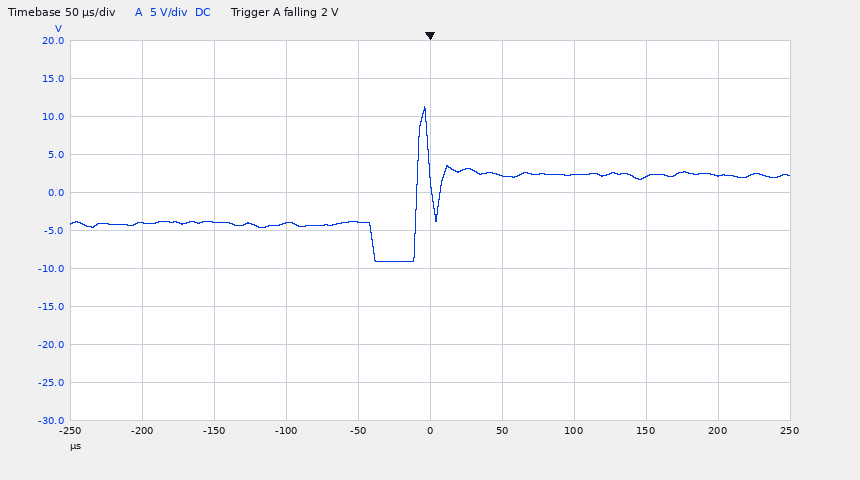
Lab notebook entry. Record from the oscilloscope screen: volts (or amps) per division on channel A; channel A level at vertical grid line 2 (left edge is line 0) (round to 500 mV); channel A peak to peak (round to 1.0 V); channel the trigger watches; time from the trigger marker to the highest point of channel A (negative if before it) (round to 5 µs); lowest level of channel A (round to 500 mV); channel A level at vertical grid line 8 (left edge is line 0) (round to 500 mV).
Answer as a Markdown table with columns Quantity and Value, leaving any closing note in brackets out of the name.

| Quantity | Value |
|---|---|
| volts (or amps) per division on channel A | 5 V |
| channel A level at vertical grid line 2 (left edge is line 0) | -4.0 V |
| channel A peak to peak | 20.0 V |
| channel the trigger watches | channel A |
| time from the trigger marker to the highest point of channel A (negative if before it) | -5 µs |
| lowest level of channel A | -9.0 V |
| channel A level at vertical grid line 8 (left edge is line 0) | 2.0 V |
